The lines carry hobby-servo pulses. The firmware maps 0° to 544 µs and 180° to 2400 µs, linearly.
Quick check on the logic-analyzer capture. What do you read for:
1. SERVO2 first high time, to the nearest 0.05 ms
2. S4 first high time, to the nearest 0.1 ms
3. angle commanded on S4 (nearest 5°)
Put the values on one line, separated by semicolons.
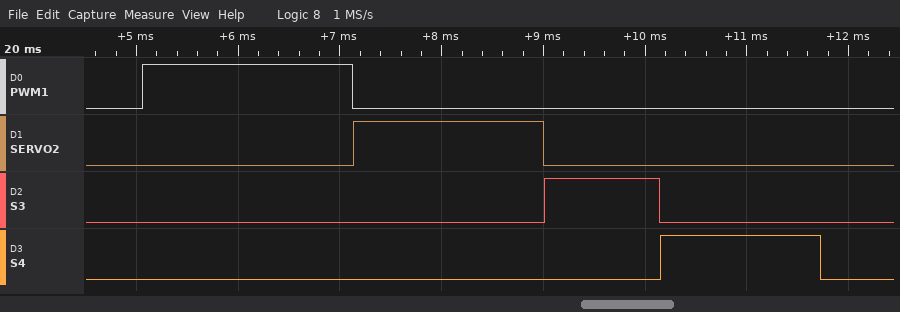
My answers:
1.85 ms; 1.6 ms; 100°
